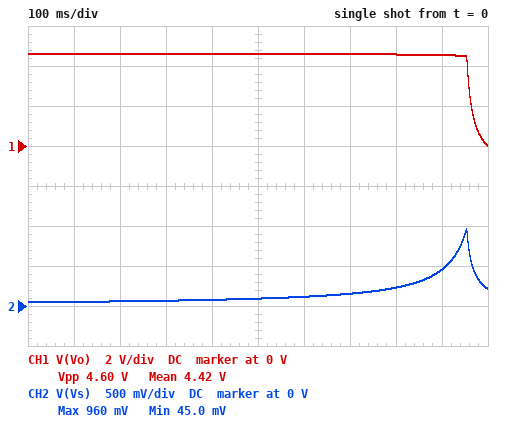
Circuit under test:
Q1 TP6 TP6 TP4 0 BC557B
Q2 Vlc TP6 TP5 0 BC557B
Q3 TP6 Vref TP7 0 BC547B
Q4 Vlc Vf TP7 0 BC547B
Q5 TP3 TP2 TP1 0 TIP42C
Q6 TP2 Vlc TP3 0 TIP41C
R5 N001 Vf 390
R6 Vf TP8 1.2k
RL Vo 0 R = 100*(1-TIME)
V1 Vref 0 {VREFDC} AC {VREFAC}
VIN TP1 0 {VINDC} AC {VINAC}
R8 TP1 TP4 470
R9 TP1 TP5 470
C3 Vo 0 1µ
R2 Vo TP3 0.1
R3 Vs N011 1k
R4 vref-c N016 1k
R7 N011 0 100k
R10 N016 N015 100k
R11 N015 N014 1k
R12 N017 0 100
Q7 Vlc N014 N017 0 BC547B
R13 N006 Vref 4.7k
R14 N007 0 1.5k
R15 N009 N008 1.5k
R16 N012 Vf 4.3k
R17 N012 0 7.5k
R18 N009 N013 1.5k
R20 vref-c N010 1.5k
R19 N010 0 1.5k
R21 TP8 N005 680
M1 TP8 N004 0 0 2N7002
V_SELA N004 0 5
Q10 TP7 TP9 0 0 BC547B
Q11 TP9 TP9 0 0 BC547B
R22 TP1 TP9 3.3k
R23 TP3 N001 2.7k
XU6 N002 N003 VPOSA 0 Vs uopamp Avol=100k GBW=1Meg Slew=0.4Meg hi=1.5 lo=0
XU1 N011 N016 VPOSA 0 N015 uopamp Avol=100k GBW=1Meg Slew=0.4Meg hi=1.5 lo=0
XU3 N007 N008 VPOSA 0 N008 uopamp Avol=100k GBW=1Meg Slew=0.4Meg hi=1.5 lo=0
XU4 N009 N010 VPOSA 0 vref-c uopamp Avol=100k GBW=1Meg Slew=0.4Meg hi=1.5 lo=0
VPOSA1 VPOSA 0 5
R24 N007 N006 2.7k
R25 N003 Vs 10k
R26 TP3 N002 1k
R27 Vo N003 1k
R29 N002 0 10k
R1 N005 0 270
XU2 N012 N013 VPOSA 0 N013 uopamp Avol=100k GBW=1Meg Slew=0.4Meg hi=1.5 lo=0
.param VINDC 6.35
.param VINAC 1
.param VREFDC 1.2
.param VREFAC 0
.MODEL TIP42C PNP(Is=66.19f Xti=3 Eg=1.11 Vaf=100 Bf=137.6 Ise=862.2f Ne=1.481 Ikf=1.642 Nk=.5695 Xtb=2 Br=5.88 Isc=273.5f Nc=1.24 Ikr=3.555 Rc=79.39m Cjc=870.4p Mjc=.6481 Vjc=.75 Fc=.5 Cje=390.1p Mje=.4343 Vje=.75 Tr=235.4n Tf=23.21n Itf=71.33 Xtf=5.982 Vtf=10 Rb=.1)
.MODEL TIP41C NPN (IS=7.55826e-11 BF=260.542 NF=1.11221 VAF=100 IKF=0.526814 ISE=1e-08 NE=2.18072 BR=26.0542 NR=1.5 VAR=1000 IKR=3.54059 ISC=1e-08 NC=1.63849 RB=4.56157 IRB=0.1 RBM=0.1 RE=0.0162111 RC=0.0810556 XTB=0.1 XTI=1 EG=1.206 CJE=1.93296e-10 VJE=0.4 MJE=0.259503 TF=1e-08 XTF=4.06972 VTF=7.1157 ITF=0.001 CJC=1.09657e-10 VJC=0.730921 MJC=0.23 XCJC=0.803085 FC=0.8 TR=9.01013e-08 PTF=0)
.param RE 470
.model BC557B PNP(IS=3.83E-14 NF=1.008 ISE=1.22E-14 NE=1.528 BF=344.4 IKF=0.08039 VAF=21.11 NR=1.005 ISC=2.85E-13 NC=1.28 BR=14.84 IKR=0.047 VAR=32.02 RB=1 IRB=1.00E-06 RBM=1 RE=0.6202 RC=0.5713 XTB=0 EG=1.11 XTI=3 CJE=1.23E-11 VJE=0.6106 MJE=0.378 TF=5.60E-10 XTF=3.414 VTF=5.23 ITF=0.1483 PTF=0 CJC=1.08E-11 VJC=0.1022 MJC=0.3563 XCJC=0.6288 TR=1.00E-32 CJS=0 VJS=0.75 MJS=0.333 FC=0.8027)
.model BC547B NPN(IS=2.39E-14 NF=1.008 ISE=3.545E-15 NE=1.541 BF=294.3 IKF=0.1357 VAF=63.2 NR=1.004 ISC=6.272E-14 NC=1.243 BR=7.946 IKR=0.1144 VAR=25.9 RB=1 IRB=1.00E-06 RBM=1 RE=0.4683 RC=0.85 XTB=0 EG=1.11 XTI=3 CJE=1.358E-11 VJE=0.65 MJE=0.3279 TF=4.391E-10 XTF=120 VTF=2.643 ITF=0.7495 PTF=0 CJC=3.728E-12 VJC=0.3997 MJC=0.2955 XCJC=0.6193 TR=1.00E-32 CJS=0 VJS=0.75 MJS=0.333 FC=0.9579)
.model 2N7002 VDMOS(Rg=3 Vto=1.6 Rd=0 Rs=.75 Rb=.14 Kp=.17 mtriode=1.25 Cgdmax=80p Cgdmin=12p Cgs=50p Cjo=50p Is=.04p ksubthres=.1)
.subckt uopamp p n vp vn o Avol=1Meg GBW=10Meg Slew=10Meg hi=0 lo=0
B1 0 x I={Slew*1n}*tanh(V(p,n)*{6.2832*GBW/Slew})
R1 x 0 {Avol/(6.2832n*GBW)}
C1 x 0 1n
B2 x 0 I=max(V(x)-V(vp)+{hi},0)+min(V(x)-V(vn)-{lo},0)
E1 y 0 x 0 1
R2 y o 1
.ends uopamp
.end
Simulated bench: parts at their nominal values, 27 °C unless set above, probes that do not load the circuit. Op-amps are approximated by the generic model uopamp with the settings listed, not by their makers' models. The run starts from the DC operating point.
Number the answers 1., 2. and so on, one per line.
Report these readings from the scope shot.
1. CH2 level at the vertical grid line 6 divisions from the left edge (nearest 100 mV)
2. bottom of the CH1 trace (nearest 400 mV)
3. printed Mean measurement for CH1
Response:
1. 100 mV
2. 0 V
3. 4.42 V
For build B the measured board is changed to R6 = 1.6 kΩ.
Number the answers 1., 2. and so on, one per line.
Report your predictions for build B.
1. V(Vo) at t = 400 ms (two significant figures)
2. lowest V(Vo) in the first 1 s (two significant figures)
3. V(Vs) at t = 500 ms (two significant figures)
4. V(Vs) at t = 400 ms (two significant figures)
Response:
1. 3.8 V
2. -2.1 mV
3. 77 mV
4. 64 mV
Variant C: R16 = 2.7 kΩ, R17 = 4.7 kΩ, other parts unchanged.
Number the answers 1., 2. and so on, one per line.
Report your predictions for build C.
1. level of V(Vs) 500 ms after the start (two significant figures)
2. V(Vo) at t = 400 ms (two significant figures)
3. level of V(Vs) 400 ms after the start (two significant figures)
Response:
1. 96 mV
2. 4.8 V
3. 80 mV
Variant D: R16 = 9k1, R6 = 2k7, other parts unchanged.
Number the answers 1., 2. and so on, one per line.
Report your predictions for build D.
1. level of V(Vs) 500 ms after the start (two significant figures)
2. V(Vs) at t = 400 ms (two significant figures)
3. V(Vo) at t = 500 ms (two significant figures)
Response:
1. 56 mV
2. 47 mV
3. 2.8 V
